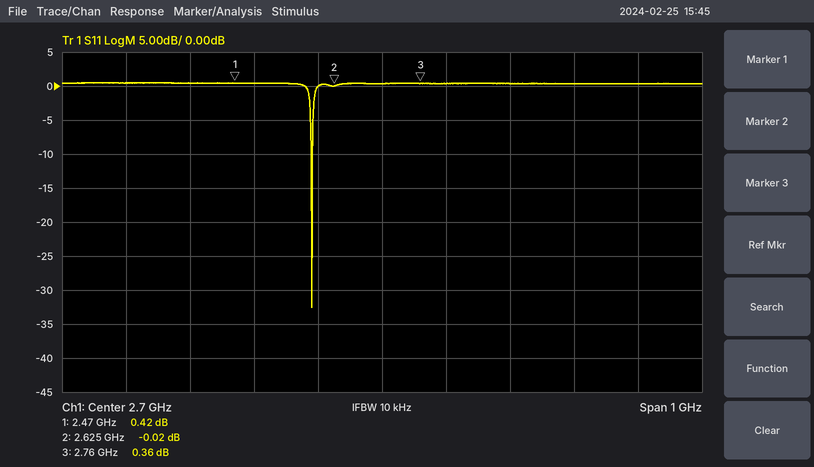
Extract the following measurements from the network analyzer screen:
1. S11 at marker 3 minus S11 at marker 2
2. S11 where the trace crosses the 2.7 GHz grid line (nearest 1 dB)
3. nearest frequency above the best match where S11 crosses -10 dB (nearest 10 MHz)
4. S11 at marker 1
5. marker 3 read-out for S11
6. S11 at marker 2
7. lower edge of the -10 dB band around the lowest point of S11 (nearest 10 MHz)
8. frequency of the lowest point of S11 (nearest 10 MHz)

0.38 dB
0 dB
2.59 GHz
0.42 dB
0.36 dB
-0.02 dB
2.59 GHz
2.59 GHz
